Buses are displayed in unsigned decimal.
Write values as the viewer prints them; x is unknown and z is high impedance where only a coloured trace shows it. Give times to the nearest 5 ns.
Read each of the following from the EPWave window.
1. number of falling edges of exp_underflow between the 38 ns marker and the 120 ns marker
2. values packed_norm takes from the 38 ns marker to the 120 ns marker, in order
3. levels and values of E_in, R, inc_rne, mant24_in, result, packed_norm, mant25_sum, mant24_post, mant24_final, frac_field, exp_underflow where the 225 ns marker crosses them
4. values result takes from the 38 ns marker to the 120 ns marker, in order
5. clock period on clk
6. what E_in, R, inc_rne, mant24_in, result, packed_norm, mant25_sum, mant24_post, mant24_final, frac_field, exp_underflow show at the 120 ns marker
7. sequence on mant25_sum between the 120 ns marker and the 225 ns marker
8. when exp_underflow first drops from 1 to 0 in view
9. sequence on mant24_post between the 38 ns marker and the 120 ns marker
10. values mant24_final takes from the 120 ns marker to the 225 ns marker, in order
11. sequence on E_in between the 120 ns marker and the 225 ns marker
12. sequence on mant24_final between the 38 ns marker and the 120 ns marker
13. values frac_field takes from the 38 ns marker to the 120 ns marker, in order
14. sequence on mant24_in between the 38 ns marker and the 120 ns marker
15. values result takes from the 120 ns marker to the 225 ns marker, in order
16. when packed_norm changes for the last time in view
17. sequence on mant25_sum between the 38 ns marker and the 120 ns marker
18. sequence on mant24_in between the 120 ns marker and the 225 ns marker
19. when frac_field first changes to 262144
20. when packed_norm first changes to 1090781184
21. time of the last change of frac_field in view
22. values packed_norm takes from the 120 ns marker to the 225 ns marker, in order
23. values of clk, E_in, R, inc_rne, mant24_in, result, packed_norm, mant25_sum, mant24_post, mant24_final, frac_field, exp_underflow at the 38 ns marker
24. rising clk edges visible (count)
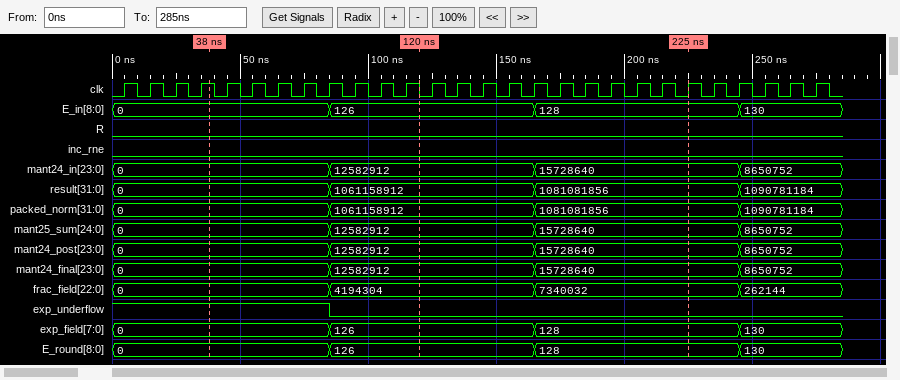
1
0, 1061158912
E_in=128, R=0, inc_rne=0, mant24_in=15728640, result=1081081856, packed_norm=1081081856, mant25_sum=15728640, mant24_post=15728640, mant24_final=15728640, frac_field=7340032, exp_underflow=0
0, 1061158912
10 ns
E_in=126, R=0, inc_rne=0, mant24_in=12582912, result=1061158912, packed_norm=1061158912, mant25_sum=12582912, mant24_post=12582912, mant24_final=12582912, frac_field=4194304, exp_underflow=0
12582912, 15728640
85 ns
0, 12582912
12582912, 15728640
126, 128
0, 12582912
0, 4194304
0, 12582912
1061158912, 1081081856
245 ns
0, 12582912
12582912, 15728640
245 ns
245 ns
245 ns
1061158912, 1081081856
clk=1, E_in=0, R=0, inc_rne=0, mant24_in=0, result=0, packed_norm=0, mant25_sum=0, mant24_post=0, mant24_final=0, frac_field=0, exp_underflow=1
28
